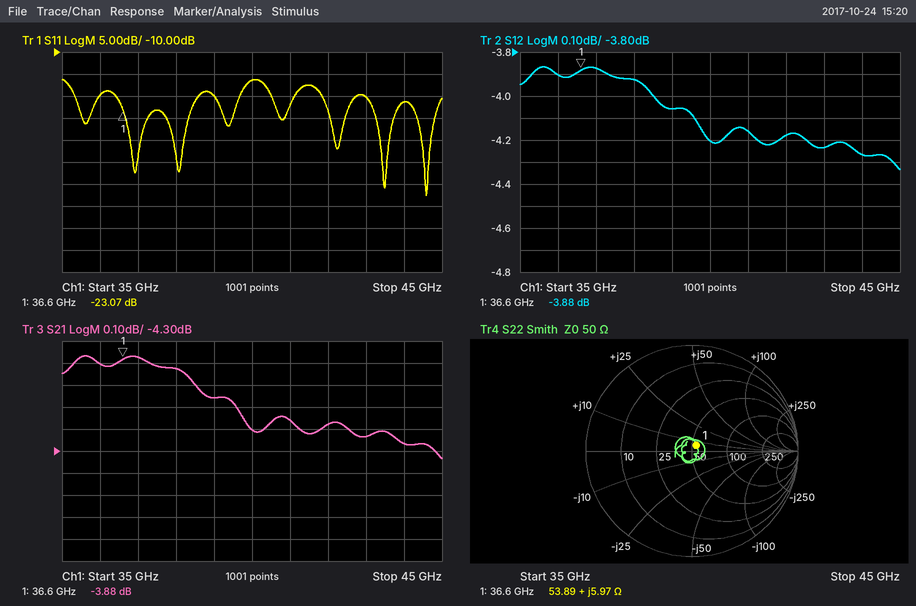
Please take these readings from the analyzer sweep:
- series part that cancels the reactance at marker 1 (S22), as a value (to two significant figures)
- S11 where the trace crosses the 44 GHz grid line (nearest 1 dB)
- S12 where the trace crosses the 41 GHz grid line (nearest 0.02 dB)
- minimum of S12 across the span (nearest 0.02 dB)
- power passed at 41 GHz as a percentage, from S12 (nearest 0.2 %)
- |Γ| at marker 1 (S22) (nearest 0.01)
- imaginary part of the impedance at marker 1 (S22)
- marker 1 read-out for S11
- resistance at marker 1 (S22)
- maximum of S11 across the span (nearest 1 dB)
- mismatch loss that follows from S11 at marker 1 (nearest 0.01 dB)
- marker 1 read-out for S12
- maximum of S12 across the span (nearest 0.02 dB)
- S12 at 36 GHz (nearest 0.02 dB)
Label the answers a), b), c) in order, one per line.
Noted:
a) 730 fF
b) -21 dB
c) -4.16 dB
d) -4.34 dB
e) 38.4 %
f) 0.07
g) +5.97 Ω
h) -23.07 dB
i) 53.89 Ω
j) -16 dB
k) 0.02 dB
l) -3.88 dB
m) -3.86 dB
n) -3.90 dB
